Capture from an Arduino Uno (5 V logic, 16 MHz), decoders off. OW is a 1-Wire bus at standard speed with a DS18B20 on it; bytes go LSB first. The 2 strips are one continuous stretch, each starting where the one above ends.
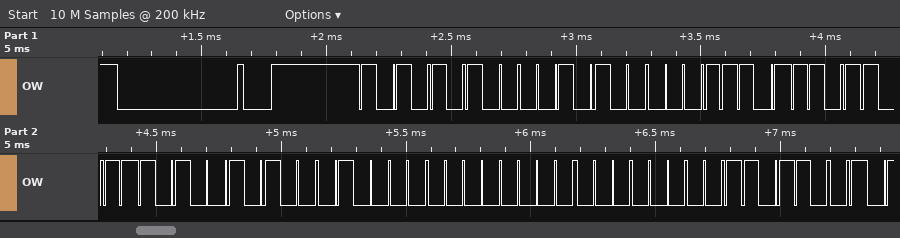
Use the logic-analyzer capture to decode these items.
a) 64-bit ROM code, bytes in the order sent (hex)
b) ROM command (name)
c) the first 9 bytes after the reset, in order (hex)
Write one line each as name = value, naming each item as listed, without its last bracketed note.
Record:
64-bit ROM code, bytes in the order sent = 28 B8 DB A5 08 00 00 9B
ROM command = Match ROM
the first 9 bytes after the reset, in order = 55 28 B8 DB A5 08 00 00 9B
